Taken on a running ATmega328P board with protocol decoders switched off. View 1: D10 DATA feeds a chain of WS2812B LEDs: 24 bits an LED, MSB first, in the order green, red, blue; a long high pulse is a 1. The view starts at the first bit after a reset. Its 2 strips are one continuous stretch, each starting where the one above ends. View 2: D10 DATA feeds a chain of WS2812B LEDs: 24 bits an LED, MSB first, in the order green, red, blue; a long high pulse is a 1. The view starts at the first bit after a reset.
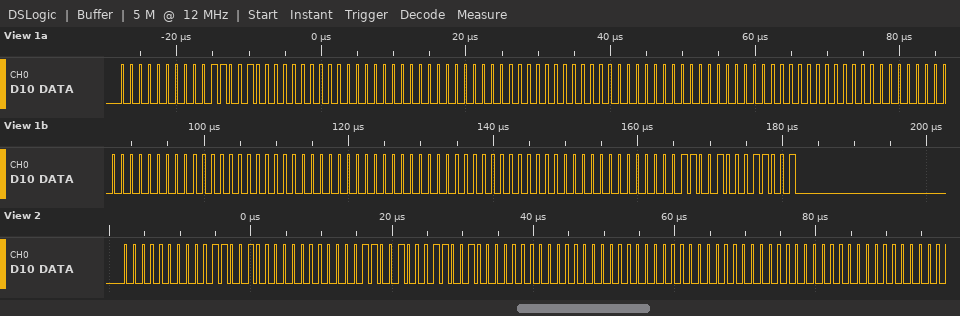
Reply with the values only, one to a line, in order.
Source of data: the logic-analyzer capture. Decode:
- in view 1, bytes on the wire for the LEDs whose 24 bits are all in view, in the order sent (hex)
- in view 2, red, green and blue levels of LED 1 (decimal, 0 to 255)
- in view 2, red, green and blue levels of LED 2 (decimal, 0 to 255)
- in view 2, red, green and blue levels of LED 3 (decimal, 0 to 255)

00 32 00 00 00 00 00 00 00 00 00 00 00 00 00 00 00 00 00 19 19
50, 0, 0
25, 25, 0
0, 0, 0
